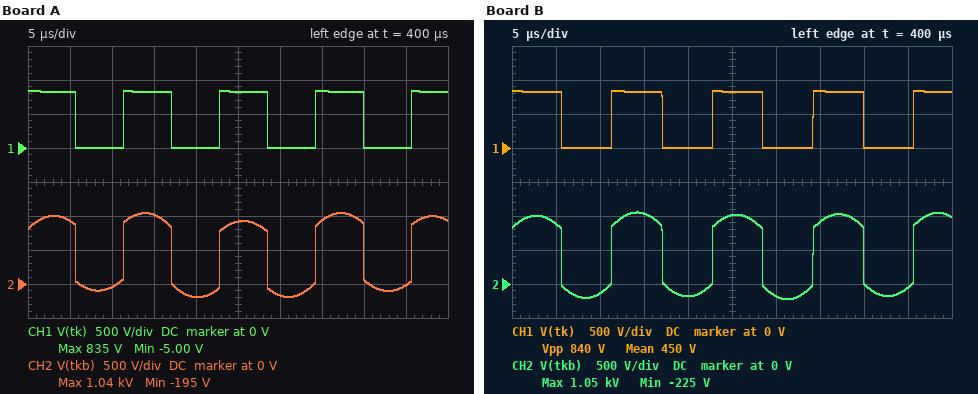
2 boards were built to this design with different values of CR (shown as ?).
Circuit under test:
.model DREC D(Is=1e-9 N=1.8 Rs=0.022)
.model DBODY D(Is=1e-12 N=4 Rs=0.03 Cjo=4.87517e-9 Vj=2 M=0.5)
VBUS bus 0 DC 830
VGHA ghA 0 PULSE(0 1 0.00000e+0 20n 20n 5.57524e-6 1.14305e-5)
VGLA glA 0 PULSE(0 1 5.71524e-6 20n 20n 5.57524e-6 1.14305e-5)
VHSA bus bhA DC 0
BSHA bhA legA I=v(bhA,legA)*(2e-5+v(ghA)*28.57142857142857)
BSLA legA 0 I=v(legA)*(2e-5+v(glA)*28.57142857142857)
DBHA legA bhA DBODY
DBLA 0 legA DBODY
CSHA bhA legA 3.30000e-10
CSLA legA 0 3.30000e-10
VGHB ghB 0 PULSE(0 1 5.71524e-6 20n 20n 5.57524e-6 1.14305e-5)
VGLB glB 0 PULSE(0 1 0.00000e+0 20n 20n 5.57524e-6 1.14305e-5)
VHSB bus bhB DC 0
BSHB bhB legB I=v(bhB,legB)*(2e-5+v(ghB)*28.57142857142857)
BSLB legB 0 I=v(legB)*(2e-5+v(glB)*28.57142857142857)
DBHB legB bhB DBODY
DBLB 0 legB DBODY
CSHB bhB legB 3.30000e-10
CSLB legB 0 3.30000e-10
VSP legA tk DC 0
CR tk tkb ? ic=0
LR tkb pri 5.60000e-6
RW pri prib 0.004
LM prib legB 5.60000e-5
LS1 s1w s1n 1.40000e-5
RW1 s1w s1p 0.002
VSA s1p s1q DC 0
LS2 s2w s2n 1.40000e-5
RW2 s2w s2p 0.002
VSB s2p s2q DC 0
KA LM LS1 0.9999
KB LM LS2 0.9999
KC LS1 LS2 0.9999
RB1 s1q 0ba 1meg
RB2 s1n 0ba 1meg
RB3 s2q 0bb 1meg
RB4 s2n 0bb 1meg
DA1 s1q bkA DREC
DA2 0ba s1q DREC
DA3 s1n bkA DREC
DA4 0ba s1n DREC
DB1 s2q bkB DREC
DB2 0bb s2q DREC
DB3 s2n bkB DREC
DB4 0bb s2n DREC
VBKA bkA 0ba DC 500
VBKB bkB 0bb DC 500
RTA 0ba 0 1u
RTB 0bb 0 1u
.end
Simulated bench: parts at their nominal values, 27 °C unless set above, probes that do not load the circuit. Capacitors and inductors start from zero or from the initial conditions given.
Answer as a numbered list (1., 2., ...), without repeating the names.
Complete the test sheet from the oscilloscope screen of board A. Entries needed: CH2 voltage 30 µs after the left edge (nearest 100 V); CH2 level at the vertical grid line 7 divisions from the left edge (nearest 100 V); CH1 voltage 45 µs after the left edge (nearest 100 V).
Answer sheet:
1. -200 V
2. 900 V
3. 0 V
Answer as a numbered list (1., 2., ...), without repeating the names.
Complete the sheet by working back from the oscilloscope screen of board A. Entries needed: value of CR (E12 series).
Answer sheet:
1. 390 nF
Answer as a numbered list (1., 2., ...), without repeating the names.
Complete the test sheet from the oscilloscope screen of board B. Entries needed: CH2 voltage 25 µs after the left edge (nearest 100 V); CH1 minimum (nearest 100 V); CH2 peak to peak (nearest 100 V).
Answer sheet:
1. 1.0 kV
2. 0 V
3. 1.3 kV
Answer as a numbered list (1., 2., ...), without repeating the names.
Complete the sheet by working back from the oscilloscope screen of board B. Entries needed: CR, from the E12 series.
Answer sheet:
1. 330 nF
